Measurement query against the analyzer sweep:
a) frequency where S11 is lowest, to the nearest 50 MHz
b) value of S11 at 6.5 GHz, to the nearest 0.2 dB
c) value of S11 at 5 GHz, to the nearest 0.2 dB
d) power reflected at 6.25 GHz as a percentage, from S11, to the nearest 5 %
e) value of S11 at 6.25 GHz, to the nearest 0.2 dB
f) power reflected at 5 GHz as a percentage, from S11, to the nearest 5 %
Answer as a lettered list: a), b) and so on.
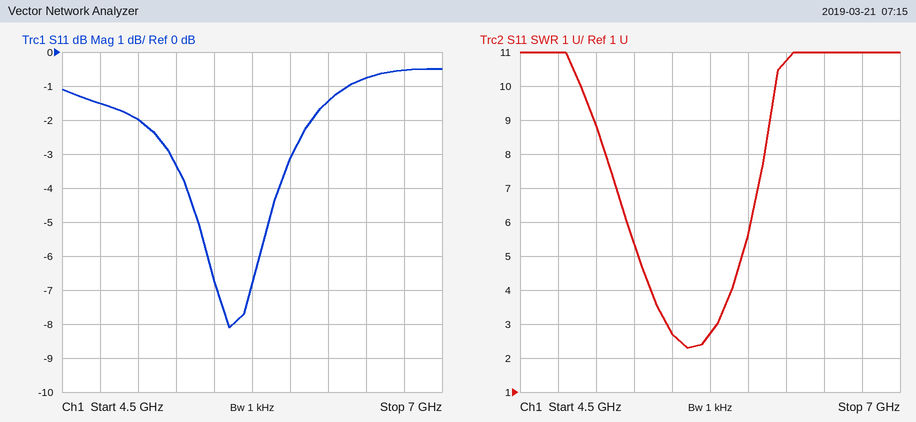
a) 5.60 GHz
b) -0.8 dB
c) -2.0 dB
d) 70 %
e) -1.4 dB
f) 65 %
